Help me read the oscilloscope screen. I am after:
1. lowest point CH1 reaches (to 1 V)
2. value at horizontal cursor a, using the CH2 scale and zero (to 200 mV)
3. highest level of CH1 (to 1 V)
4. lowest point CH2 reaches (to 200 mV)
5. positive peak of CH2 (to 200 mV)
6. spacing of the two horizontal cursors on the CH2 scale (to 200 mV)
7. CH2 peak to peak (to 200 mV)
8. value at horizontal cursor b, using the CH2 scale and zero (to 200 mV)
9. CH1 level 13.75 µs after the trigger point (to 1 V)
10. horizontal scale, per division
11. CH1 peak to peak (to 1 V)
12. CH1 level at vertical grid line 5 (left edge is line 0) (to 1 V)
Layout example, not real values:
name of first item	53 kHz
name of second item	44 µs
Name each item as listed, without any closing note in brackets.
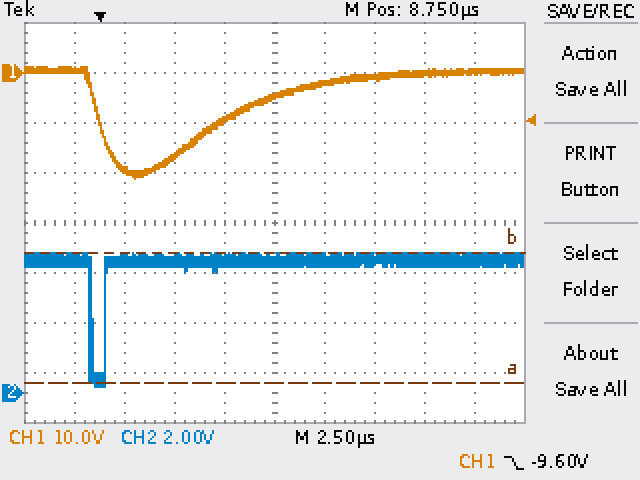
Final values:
lowest point CH1 reaches	-21 V
value at horizontal cursor a, using the CH2 scale and zero	400 mV
highest level of CH1	1 V
lowest point CH2 reaches	200 mV
positive peak of CH2	5.6 V
spacing of the two horizontal cursors on the CH2 scale	5.2 V
CH2 peak to peak	5.4 V
value at horizontal cursor b, using the CH2 scale and zero	5.6 V
CH1 level 13.75 µs after the trigger point	-1 V
horizontal scale, per division	2.5 µs
CH1 peak to peak	22 V
CH1 level at vertical grid line 5 (left edge is line 0)	-5 V
